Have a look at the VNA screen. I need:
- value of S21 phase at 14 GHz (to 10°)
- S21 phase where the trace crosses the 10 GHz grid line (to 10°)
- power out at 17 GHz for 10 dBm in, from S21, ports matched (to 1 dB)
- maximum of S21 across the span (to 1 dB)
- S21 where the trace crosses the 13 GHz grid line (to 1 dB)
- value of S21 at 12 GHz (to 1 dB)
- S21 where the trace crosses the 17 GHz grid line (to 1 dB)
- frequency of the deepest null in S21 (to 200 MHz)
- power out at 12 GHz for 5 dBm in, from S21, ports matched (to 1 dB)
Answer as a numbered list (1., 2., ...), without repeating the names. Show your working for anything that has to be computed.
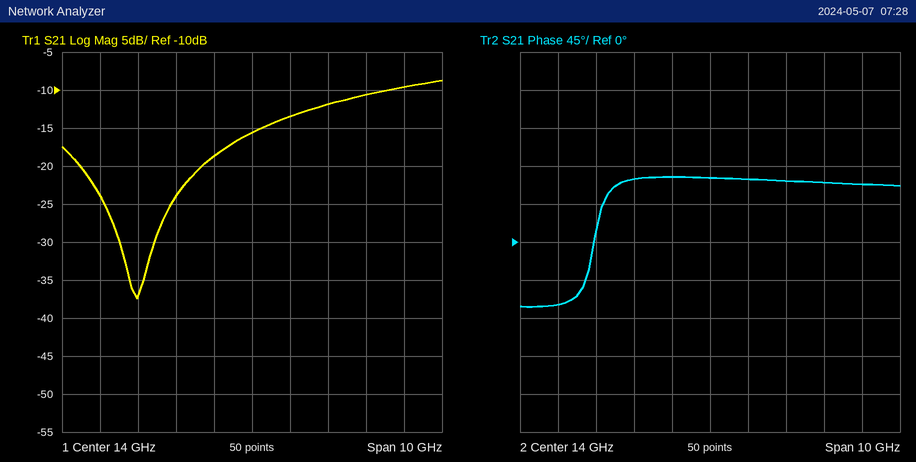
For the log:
1. 80°
2. -70°
3. 10 dBm + (-11 dB) = -1 dBm
4. -9 dB
5. -19 dB
6. -24 dB
7. -11 dB
8. 11.0 GHz
9. 5 dBm + (-24 dB) = -19 dBm
